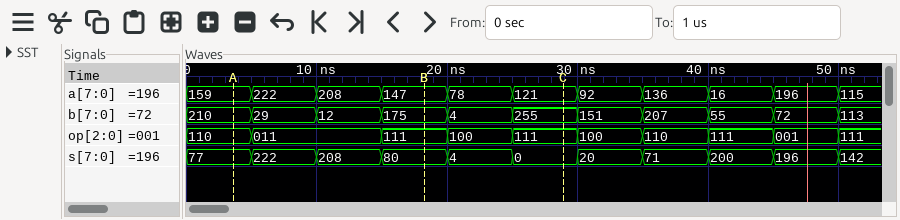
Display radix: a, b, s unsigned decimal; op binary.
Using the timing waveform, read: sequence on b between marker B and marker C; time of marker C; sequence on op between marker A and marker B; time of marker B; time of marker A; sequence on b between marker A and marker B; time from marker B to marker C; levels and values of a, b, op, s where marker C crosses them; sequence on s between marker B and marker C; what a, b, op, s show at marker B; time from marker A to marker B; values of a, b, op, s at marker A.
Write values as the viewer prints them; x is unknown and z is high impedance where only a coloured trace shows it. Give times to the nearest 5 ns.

175, 4, 255
30 ns
110, 011, 111
20 ns
5 ns
210, 29, 12, 175
10 ns
a=121, b=255, op=111, s=0
80, 4, 0
a=147, b=175, op=111, s=80
15 ns
a=159, b=210, op=110, s=77
